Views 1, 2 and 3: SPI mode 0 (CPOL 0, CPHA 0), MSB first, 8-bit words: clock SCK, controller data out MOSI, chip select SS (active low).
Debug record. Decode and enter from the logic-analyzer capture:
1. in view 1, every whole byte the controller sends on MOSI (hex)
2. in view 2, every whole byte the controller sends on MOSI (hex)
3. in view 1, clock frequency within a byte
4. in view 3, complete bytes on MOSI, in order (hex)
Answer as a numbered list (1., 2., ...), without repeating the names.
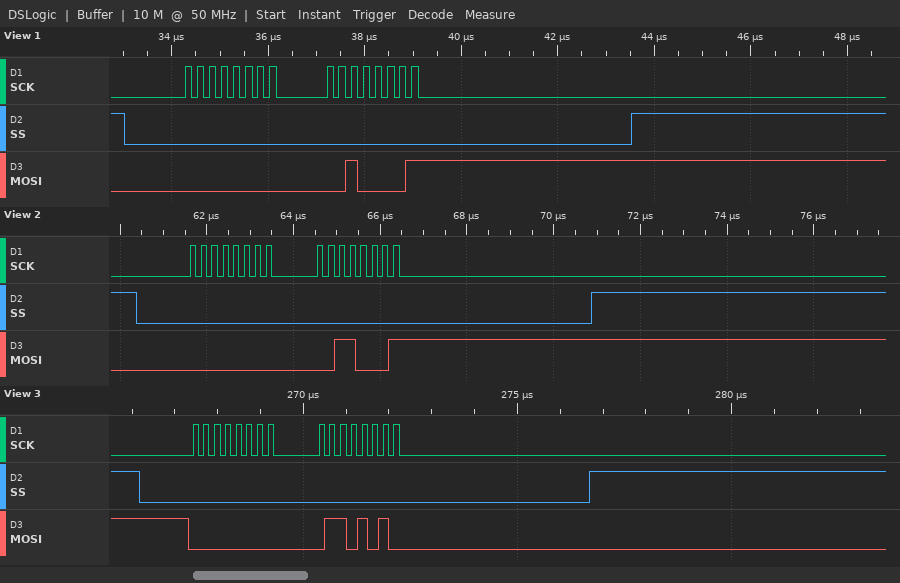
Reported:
1. 00 21
2. 00 31
3. 4 MHz
4. 00 6A
